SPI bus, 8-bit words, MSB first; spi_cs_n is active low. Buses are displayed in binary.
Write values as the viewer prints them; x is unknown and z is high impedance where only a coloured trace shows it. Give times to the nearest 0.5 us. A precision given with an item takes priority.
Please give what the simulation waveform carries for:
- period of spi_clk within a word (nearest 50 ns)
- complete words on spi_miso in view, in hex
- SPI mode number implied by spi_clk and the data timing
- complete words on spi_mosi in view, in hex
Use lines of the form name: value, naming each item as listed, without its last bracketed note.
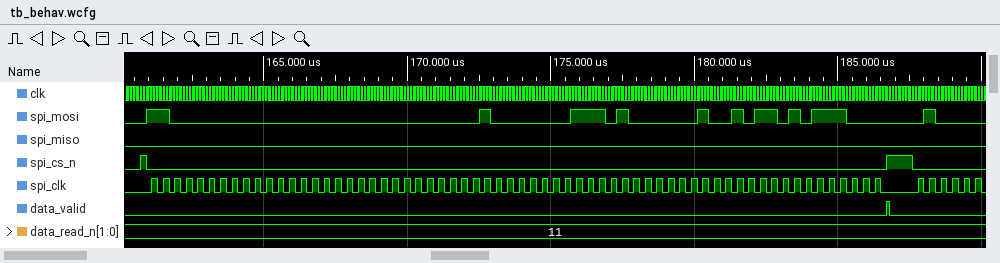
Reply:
period of spi_clk within a word: 400 ns
complete words on spi_miso in view, in hex: 00, 00, 00, 00, 00, 00, 00, 00
SPI mode number implied by spi_clk and the data timing: 0
complete words on spi_mosi in view, in hex: C0, 00, 00, 04, 07, 40, 96, B8
